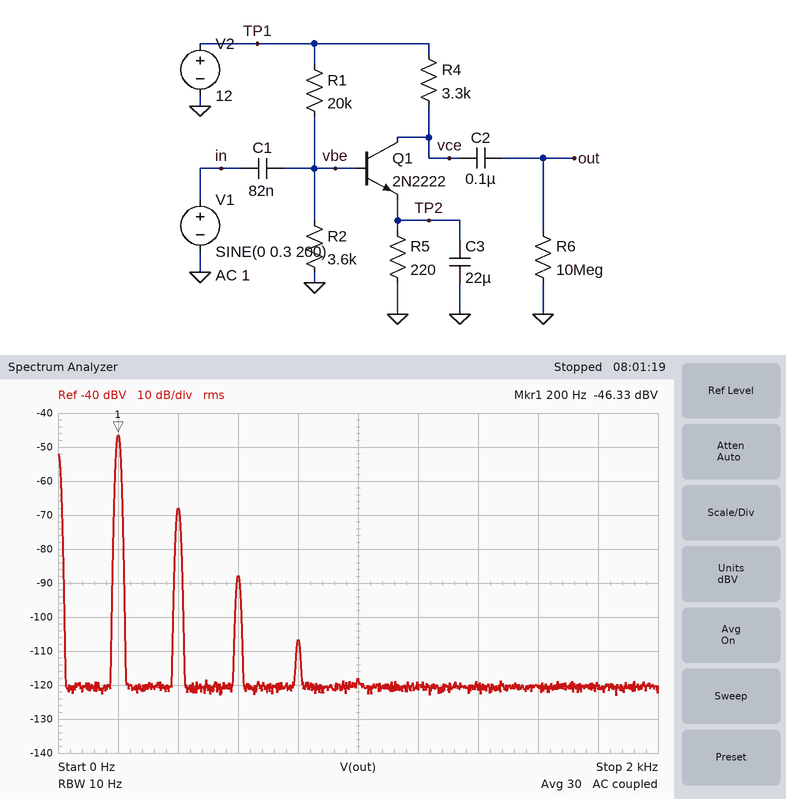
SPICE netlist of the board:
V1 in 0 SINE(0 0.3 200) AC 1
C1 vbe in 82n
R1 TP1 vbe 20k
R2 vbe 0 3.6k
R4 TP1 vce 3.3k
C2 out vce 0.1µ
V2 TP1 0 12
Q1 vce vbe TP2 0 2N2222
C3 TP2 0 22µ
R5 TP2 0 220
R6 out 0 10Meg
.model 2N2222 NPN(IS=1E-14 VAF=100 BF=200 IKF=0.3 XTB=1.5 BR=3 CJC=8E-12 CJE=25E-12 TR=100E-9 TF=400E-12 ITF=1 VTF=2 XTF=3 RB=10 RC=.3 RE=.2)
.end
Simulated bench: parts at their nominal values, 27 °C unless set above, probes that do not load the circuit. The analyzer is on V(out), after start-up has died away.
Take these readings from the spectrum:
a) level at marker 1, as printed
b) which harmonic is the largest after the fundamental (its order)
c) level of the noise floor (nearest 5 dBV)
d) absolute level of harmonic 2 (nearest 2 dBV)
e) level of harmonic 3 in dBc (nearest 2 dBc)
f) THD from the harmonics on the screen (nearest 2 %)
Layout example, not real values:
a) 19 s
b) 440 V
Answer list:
a) -46.33 dBV
b) 2
c) -120 dBV
d) -68 dBV
e) -42 dBc
f) 8 %
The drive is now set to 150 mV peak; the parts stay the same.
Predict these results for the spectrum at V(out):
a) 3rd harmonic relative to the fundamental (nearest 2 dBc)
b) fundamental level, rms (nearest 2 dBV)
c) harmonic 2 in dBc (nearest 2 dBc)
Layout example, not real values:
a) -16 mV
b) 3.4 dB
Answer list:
a) -54 dBc
b) -52 dBV
c) -28 dBc
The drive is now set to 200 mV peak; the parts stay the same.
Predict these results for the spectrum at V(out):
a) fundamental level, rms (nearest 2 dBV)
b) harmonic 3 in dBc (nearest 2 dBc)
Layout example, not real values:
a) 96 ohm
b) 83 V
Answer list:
a) -50 dBV
b) -48 dBc
